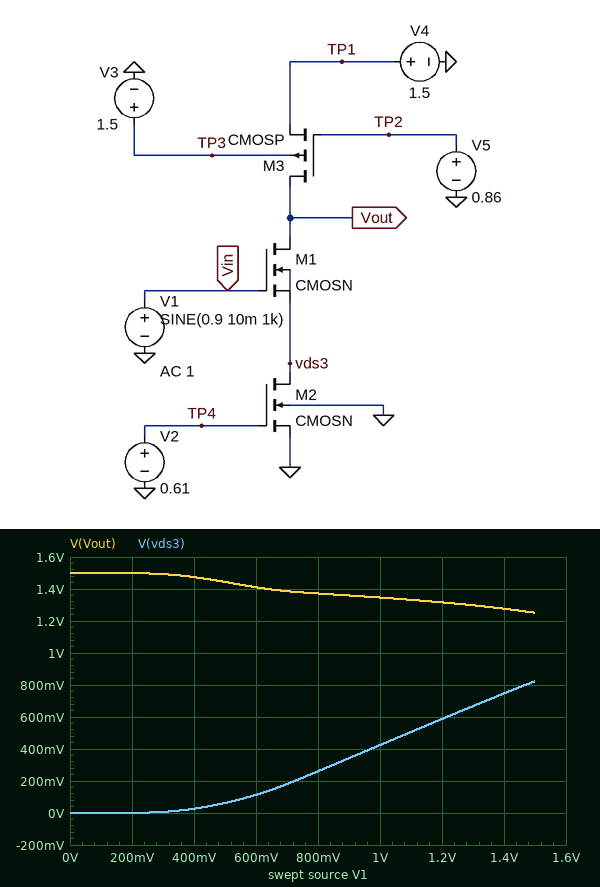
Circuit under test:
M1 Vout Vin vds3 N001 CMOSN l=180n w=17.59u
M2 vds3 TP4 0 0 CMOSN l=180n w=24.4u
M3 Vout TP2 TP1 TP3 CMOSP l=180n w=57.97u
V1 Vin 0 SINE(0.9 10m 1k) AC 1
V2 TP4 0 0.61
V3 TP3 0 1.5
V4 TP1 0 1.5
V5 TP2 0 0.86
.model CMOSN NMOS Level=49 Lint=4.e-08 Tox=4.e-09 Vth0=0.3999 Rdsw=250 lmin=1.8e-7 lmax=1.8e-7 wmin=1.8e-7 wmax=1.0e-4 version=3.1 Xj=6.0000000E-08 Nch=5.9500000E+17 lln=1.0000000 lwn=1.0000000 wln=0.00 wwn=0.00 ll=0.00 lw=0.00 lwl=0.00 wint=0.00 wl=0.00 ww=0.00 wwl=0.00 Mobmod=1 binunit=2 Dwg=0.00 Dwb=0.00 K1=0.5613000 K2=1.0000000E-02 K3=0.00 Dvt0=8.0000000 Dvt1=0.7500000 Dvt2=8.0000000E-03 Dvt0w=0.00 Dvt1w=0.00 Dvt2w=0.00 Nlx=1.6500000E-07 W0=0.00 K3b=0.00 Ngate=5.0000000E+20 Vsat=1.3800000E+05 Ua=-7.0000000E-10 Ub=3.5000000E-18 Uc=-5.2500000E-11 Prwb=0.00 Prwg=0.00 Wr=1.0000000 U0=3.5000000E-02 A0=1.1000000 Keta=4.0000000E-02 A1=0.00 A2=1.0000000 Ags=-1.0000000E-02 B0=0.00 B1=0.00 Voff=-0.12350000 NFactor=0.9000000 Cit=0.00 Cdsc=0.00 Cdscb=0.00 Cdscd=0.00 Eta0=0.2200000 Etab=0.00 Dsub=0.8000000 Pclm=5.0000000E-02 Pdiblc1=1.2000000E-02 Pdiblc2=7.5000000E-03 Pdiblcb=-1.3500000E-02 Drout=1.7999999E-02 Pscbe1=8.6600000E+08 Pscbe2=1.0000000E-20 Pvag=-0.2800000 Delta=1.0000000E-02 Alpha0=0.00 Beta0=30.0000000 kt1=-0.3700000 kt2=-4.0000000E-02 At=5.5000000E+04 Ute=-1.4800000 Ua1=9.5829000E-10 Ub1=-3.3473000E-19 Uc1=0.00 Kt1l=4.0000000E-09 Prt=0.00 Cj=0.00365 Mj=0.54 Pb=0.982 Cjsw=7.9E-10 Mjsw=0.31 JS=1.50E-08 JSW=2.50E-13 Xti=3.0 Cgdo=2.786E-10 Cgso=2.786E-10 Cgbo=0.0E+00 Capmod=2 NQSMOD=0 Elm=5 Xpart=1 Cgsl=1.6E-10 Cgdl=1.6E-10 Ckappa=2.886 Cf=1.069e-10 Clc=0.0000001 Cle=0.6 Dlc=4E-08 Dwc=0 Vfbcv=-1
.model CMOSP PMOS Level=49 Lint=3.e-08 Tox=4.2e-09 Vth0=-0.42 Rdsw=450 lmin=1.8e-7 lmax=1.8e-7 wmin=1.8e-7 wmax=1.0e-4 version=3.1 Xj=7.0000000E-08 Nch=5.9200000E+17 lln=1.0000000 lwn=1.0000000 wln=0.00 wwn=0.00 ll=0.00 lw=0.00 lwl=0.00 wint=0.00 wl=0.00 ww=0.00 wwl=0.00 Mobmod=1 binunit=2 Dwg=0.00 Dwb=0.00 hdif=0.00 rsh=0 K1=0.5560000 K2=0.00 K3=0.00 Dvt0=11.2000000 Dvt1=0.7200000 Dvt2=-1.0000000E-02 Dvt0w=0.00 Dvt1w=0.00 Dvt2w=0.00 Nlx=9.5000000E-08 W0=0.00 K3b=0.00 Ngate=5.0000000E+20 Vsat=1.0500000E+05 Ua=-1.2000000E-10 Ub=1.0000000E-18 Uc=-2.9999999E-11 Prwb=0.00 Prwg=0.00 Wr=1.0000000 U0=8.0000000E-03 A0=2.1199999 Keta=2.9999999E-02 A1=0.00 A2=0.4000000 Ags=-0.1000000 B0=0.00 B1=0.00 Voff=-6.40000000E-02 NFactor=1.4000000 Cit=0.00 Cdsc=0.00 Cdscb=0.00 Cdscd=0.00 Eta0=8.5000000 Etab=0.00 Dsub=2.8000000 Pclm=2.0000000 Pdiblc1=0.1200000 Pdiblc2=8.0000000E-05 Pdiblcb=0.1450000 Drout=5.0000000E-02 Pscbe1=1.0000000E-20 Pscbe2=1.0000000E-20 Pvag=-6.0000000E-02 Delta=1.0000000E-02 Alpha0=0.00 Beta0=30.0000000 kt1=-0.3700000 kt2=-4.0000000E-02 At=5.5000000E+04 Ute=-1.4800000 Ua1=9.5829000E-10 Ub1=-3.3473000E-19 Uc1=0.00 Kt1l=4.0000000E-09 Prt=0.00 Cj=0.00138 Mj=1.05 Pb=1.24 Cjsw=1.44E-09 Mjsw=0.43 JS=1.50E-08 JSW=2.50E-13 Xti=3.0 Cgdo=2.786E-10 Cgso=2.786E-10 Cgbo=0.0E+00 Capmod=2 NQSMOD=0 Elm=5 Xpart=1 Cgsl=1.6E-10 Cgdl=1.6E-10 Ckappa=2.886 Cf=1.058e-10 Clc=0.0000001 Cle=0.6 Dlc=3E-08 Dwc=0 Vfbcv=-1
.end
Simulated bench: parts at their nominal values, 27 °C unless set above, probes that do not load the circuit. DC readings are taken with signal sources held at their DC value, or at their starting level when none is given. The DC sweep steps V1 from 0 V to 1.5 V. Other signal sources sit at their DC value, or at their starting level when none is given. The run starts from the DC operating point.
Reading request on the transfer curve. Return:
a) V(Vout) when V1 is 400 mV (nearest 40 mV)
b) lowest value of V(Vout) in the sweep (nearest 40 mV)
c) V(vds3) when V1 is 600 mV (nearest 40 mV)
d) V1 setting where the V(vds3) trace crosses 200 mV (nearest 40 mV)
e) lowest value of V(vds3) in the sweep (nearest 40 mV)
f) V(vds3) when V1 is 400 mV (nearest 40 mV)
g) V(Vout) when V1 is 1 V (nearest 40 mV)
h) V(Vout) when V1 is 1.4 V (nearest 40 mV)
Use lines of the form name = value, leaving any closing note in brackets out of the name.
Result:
V(Vout) when V1 is 400 mV = 1.48 V
lowest value of V(Vout) in the sweep = 1.24 V
V(vds3) when V1 is 600 mV = 120 mV
V1 setting where the V(vds3) trace crosses 200 mV = 720 mV
lowest value of V(vds3) in the sweep = 0 V
V(vds3) when V1 is 400 mV = 40 mV
V(Vout) when V1 is 1 V = 1.36 V
V(Vout) when V1 is 1.4 V = 1.28 V
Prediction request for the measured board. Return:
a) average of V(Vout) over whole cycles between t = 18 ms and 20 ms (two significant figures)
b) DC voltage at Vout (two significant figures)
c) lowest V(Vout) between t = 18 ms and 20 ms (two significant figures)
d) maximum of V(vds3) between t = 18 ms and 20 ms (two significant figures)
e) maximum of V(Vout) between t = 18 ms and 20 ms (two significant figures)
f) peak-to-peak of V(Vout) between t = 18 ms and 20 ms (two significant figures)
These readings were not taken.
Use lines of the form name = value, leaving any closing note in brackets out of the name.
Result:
average of V(Vout) over whole cycles between t = 18 ms and 20 ms = 1.4 V
DC voltage at Vout = 1.4 V
lowest V(Vout) between t = 18 ms and 20 ms = 1.4 V
maximum of V(vds3) between t = 18 ms and 20 ms = 350 mV
maximum of V(Vout) between t = 18 ms and 20 ms = 1.4 V
peak-to-peak of V(Vout) between t = 18 ms and 20 ms = 2.4 mV
